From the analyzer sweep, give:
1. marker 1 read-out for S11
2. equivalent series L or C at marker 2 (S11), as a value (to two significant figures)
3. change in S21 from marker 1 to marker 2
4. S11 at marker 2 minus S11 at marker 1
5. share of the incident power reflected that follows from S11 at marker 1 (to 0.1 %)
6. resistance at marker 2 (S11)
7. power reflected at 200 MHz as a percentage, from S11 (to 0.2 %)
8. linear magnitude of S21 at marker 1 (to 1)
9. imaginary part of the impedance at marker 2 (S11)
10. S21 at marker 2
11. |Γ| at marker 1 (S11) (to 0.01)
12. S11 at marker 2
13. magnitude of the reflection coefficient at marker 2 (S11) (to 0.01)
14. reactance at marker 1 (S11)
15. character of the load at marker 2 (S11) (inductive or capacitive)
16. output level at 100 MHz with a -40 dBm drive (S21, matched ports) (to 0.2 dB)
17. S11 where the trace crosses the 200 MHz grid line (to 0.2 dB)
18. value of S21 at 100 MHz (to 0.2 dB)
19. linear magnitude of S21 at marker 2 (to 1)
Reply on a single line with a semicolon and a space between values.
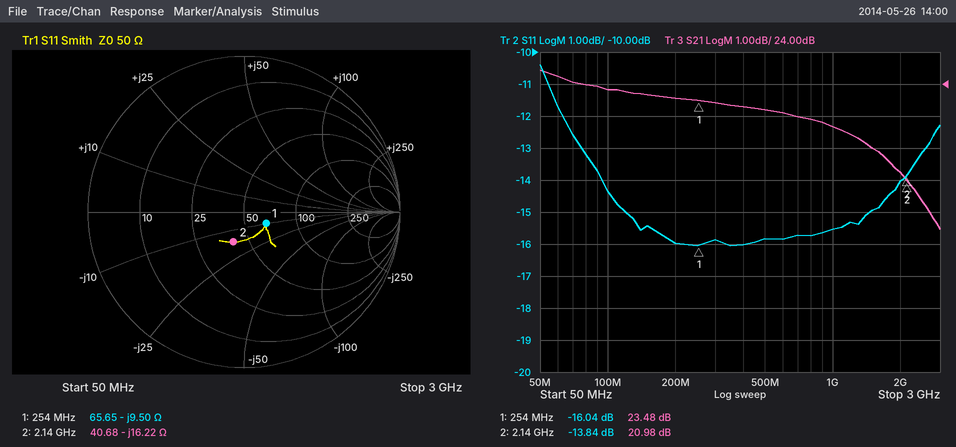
-16.04 dB; 4.6 pF; -2.50 dB; 2.20 dB; 2.5 %; 40.68 Ω; 2.6 %; 15; -16.22 Ω; 20.98 dB; 0.16; -13.84 dB; 0.20; -9.50 Ω; capacitive; -16.2 dBm; -16.0 dB; 23.8 dB; 11
